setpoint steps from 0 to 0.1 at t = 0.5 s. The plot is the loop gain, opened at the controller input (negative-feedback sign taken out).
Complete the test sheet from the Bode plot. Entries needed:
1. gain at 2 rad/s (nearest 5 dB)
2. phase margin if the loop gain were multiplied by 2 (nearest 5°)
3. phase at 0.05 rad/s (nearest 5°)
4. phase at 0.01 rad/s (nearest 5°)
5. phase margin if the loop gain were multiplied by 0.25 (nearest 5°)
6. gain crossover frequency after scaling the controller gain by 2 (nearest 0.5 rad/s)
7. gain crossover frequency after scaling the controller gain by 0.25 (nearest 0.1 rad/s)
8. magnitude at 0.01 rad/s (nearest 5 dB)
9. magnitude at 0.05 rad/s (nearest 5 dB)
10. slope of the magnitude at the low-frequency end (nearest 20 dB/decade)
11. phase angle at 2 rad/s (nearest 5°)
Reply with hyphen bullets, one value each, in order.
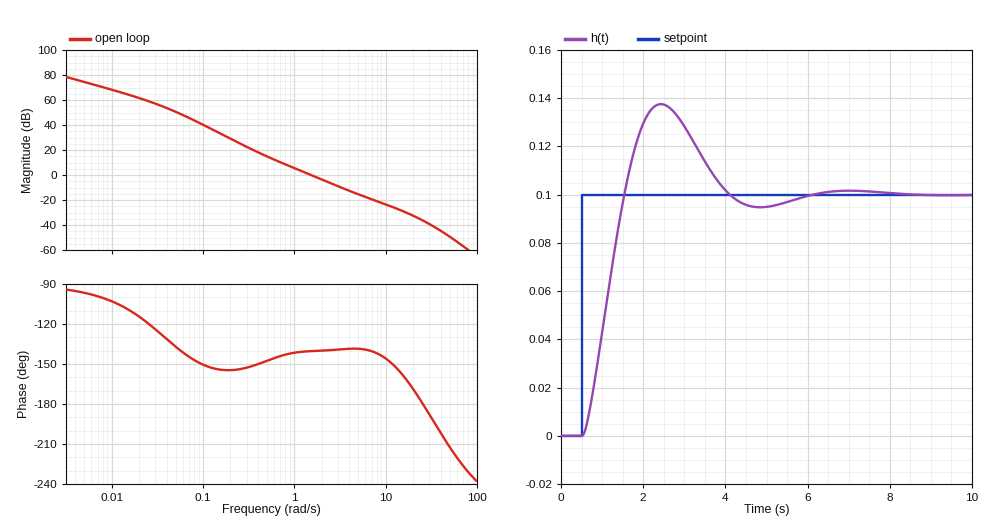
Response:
- -5 dB
- 40°
- -135°
- -105°
- 35°
- 2.5 rad/s
- 0.6 rad/s
- 70 dB
- 50 dB
- -20 dB/decade
- -140°
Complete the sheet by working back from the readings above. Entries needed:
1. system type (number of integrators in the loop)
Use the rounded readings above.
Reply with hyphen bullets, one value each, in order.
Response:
- 1
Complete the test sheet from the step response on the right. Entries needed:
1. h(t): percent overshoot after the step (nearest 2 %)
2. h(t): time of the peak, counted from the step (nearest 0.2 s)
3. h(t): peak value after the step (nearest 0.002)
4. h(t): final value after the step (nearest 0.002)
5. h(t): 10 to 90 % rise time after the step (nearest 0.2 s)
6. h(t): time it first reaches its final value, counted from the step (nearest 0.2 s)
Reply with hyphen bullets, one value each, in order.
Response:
- 38 %
- 2.0 s
- 0.138
- 0.100
- 0.8 s
- 1.0 s
